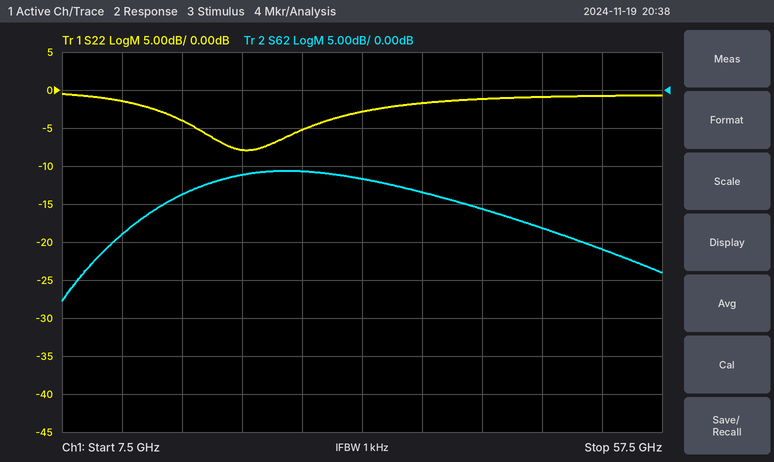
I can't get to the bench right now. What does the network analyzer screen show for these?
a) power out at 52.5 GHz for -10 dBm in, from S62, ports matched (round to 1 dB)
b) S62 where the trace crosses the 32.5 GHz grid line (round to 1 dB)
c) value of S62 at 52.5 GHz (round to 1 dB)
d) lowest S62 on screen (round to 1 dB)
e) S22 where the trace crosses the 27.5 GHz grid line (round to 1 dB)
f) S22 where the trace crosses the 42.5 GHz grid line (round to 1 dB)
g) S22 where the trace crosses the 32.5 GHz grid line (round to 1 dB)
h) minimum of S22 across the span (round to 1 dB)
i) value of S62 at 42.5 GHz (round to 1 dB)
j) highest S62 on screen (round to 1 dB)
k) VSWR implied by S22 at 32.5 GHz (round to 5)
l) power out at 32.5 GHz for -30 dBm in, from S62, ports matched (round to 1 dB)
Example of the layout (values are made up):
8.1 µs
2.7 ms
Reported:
-31 dBm
-12 dB
-21 dB
-28 dB
-5 dB
-1 dB
-3 dB
-8 dB
-16 dB
-11 dB
5
-42 dBm
